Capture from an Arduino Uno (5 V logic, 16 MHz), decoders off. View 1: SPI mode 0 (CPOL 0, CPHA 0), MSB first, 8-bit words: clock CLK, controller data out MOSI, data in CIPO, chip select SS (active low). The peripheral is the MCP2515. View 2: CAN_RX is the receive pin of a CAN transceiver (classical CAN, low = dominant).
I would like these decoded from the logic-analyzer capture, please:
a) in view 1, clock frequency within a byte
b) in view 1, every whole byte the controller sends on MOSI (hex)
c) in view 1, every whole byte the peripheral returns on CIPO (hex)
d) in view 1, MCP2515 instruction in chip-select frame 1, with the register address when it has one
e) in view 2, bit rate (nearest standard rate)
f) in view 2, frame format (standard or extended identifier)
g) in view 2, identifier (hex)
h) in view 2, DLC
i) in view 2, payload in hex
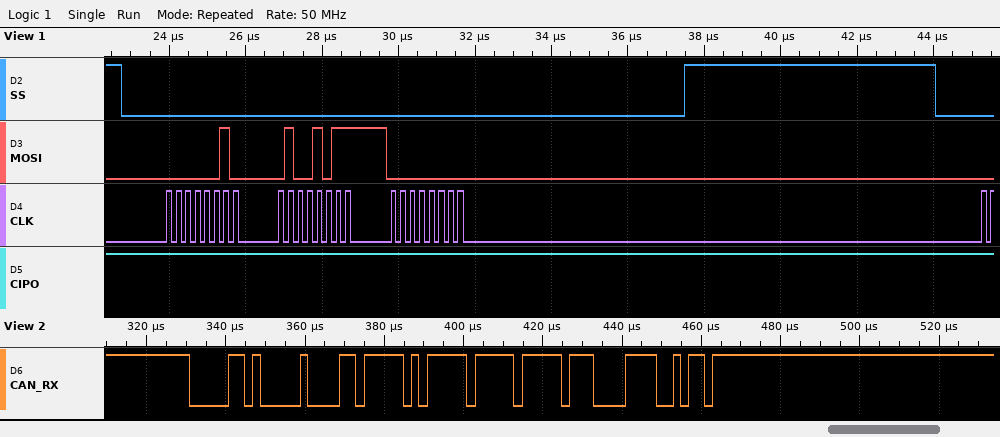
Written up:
4 MHz
02 4B 00
FF FF FF
WRITE 0x4B
500 kbit/s
standard
0x050
3
7E FF FF
